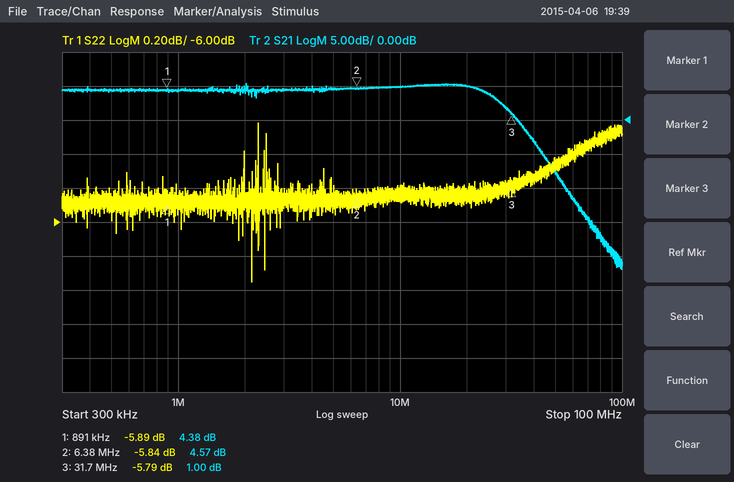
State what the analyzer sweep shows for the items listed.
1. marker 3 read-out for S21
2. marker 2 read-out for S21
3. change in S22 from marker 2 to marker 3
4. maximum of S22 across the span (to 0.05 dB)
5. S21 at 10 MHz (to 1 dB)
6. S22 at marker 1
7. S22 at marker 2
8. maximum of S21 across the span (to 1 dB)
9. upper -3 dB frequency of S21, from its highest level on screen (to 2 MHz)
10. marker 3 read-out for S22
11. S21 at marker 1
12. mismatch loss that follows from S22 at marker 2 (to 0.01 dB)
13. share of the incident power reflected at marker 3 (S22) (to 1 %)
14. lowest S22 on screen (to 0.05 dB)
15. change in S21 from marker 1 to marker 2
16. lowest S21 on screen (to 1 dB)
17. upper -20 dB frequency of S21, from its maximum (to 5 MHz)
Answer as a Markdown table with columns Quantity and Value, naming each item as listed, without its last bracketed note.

| Quantity | Value |
|---|---|
| marker 3 read-out for S21 | 1.00 dB |
| marker 2 read-out for S21 | 4.57 dB |
| change in S22 from marker 2 to marker 3 | 0.05 dB |
| maximum of S22 across the span | -5.40 dB |
| S21 at 10 MHz | 5 dB |
| S22 at marker 1 | -5.89 dB |
| S22 at marker 2 | -5.84 dB |
| maximum of S21 across the span | 5 dB |
| upper -3 dB frequency of S21, from its highest level on screen | 28 MHz |
| marker 3 read-out for S22 | -5.79 dB |
| S21 at marker 1 | 4.38 dB |
| mismatch loss that follows from S22 at marker 2 | 1.31 dB |
| share of the incident power reflected at marker 3 (S22) | 26 % |
| lowest S22 on screen | -6.35 dB |
| change in S21 from marker 1 to marker 2 | 0.19 dB |
| lowest S21 on screen | -22 dB |
| upper -20 dB frequency of S21, from its maximum | 70 MHz |
